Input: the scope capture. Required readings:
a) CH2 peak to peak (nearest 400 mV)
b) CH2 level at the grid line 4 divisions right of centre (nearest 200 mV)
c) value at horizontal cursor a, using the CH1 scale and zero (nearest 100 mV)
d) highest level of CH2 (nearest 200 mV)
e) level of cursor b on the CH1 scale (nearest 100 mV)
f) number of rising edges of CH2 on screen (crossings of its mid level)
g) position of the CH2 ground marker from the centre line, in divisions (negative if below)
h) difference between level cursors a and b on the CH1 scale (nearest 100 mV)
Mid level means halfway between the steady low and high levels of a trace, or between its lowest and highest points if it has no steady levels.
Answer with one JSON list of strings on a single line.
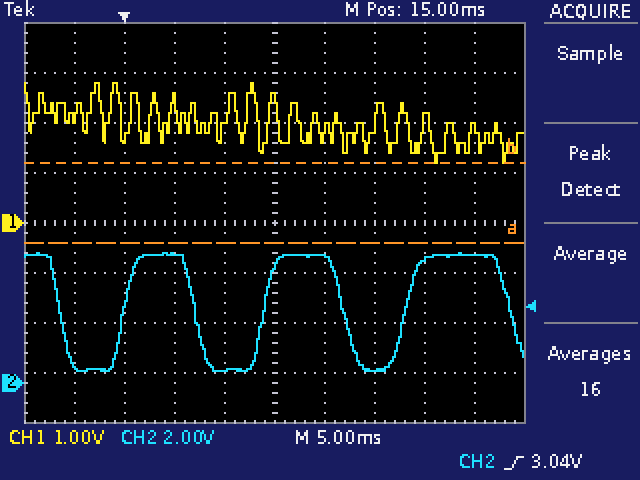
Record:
["4.8 V", "5.2 V", "-400 mV", "5.2 V", "1.2 V", "3", "-3.2 div", "1.6 V"]
